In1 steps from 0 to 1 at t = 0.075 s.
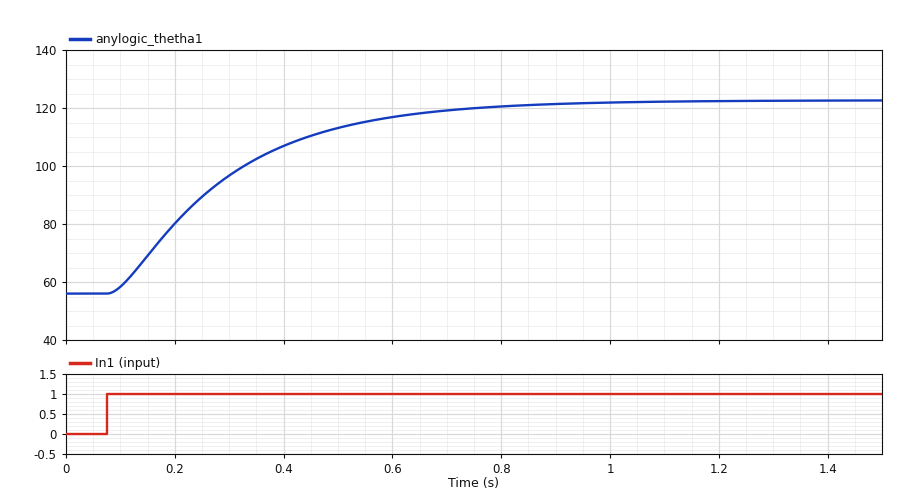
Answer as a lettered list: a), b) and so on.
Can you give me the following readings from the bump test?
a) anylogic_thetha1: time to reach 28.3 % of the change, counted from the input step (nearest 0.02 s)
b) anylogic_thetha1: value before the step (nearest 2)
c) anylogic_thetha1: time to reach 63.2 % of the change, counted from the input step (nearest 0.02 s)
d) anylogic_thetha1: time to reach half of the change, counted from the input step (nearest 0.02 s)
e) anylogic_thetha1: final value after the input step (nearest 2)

a) 0.10 s
b) 56
c) 0.24 s
d) 0.18 s
e) 122
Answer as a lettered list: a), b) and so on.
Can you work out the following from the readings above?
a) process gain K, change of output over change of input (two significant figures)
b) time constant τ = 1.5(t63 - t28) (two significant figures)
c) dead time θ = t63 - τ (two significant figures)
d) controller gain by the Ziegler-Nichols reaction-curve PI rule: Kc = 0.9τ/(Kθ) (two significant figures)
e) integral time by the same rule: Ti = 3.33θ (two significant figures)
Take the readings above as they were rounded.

a) 66
b) 0.21 s
c) 0.030 s
d) 0.095
e) 0.100 s
